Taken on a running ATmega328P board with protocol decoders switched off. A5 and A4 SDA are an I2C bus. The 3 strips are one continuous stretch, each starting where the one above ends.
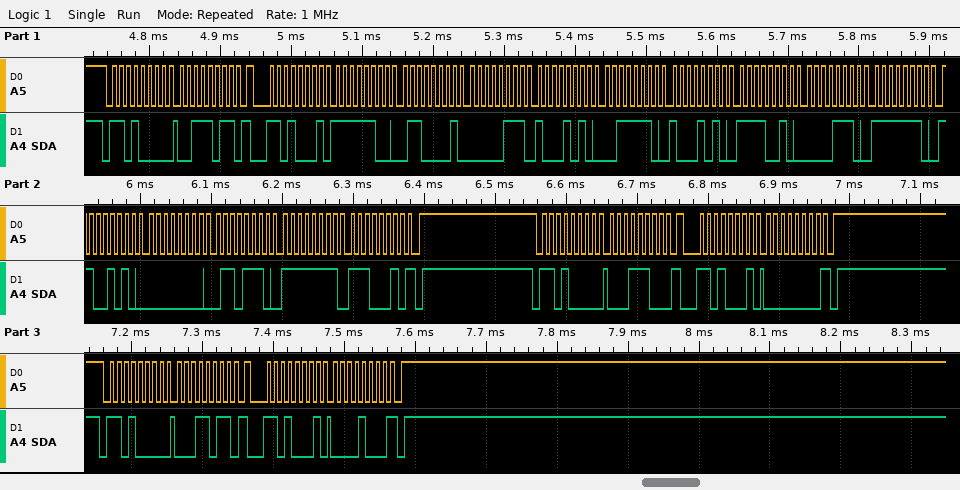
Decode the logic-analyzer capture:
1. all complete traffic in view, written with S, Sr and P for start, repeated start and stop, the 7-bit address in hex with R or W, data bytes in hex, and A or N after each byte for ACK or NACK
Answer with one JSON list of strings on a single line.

["S 68W A 3B A Sr 68R A FC A 61 A 07 A 8A A 3E A 8A A F2 A 0E A FE A CA A 00 A 6E A FF A E2 N P S 68W A 1C A Sr 68R A 00 N P S 68W A 1B A Sr 68R A 08 N P"]
